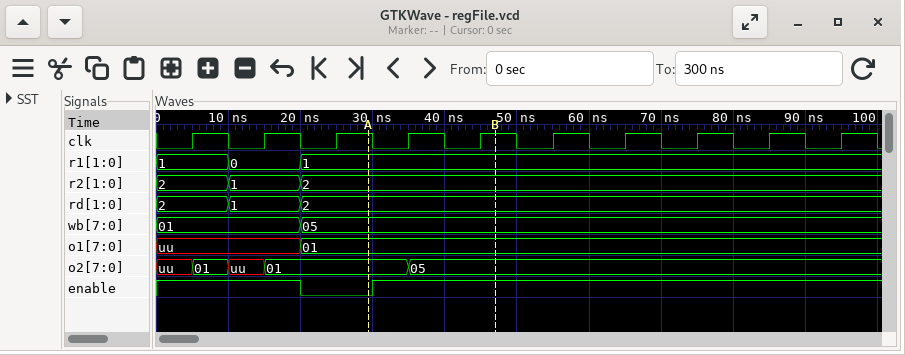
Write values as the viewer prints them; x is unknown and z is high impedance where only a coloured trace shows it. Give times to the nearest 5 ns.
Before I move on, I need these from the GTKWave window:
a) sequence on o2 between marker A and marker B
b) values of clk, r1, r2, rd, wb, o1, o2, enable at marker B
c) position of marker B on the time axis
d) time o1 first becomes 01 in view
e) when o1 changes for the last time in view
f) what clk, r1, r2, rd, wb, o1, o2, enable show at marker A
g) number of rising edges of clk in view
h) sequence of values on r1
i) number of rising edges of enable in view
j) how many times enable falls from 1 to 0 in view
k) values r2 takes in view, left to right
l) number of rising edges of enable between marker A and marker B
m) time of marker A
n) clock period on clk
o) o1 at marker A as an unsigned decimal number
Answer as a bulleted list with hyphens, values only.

- 01, 05
- clk=1, r1=1, r2=2, rd=2, wb=05, o1=01, o2=05, enable=1
- 45 ns
- 20 ns
- 20 ns
- clk=1, r1=1, r2=2, rd=2, wb=05, o1=01, o2=01, enable=0
- 10
- 1, 0, 1
- 1
- 1
- 2, 1, 2
- 1
- 30 ns
- 10 ns
- 1
